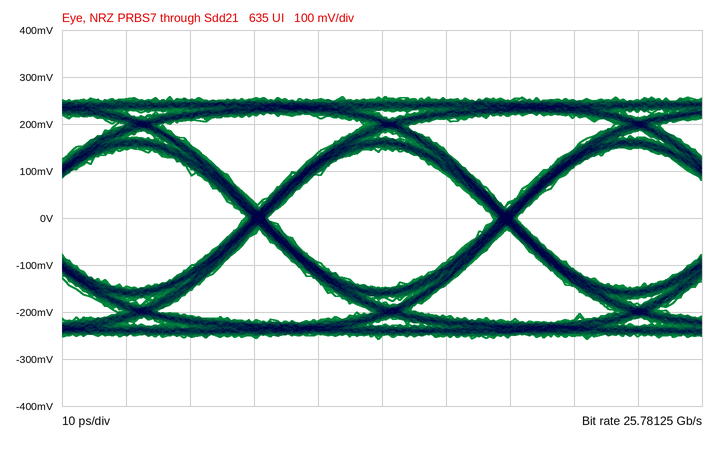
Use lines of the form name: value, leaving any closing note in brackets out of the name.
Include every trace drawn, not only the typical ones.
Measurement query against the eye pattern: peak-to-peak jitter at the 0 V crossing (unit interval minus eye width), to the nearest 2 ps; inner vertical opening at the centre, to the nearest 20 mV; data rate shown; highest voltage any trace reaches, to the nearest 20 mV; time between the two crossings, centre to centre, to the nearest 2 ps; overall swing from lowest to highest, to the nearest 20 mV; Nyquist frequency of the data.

peak-to-peak jitter at the 0 V crossing (unit interval minus eye width), to the nearest 2 ps: 4 ps
inner vertical opening at the centre, to the nearest 20 mV: 300 mV
data rate shown: 25.78125 Gb/s
highest voltage any trace reaches, to the nearest 20 mV: 260 mV
time between the two crossings, centre to centre, to the nearest 2 ps: 38 ps
overall swing from lowest to highest, to the nearest 20 mV: 520 mV
Nyquist frequency of the data: 12.89062 GHz
